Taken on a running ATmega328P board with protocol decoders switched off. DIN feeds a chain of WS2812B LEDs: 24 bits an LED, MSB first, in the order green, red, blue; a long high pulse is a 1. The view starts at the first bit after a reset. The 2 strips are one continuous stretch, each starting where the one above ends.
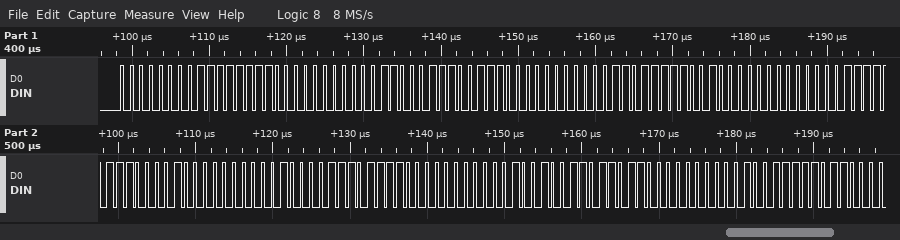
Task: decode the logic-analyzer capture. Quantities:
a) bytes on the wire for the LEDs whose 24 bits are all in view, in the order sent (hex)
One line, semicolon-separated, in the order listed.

00 FF 00 18 E7 00 1B E4 00 1E E1 00 21 DE 00 24 DB 00
